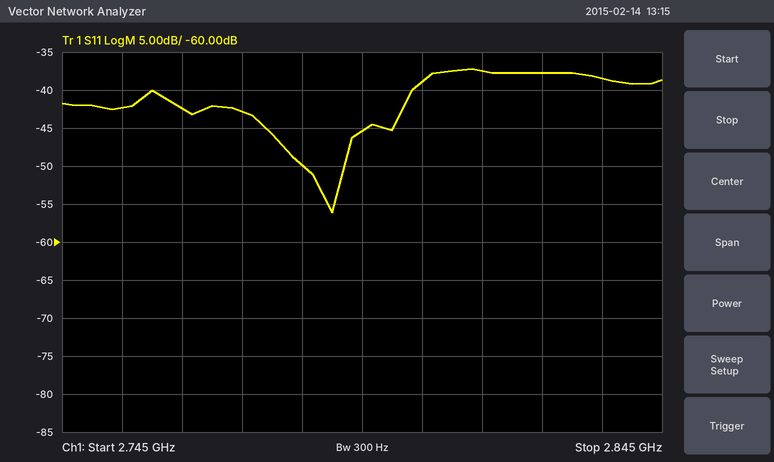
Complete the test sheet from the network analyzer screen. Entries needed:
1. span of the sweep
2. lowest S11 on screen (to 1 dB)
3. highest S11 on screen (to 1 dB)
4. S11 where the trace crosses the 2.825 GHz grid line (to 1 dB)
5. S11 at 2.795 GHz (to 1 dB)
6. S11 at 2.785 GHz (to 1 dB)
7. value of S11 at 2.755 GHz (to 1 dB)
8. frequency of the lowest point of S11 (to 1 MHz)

100 MHz
-56 dB
-37 dB
-38 dB
-45 dB
-50 dB
-42 dB
2.790 GHz
